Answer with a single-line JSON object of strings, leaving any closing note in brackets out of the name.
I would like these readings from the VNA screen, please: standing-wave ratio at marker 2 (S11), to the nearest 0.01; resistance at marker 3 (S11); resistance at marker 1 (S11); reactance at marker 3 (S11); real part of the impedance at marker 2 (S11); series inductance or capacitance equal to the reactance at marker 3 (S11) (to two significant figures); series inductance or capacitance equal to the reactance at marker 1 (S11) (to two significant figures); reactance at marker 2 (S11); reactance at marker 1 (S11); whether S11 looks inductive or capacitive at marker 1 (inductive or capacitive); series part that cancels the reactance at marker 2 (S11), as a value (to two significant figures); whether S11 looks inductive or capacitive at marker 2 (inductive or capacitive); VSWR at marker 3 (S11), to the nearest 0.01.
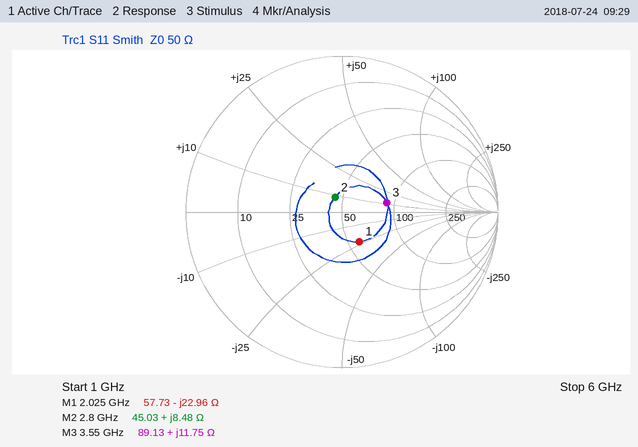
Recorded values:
{"standing-wave ratio at marker 2 (S11), to the nearest 0.01": "1.23", "resistance at marker 3": "89.13 Ω", "resistance at marker 1": "57.73 Ω", "reactance at marker 3": "+11.75 Ω", "real part of the impedance at marker 2": "45.03 Ω", "series inductance or capacitance equal to the reactance at marker 3 (S11)": "530 pH", "series inductance or capacitance equal to the reactance at marker 1 (S11)": "3.4 pF", "reactance at marker 2": "+8.48 Ω", "reactance at marker 1": "-22.96 Ω", "whether S11 looks inductive or capacitive at marker 1": "capacitive", "series part that cancels the reactance at marker 2 (S11), as a value": "6.7 pF", "whether S11 looks inductive or capacitive at marker 2": "inductive", "VSWR at marker 3 (S11), to the nearest 0.01": "1.83"}
